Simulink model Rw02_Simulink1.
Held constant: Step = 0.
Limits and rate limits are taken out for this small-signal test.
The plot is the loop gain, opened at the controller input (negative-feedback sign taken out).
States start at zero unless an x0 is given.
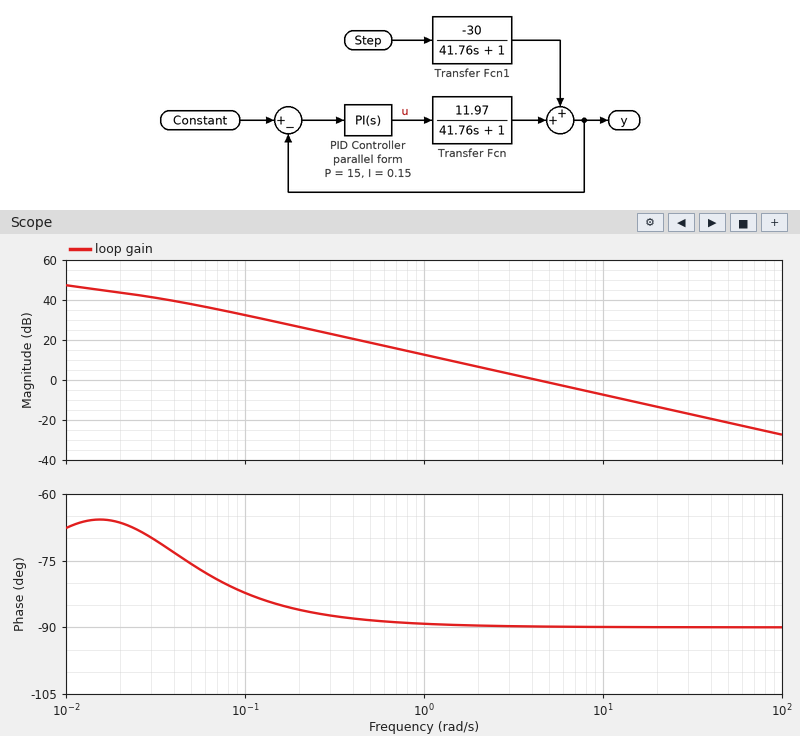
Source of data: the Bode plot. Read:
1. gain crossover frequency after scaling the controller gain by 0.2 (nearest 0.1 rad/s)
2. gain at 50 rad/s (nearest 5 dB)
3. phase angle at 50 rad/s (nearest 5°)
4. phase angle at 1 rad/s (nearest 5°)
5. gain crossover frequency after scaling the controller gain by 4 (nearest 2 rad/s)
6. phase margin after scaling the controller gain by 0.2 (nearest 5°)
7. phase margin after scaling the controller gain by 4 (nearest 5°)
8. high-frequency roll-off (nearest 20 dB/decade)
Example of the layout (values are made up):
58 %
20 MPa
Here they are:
0.9 rad/s
-20 dB
-90°
-90°
18 rad/s
90°
90°
-20 dB/decade
